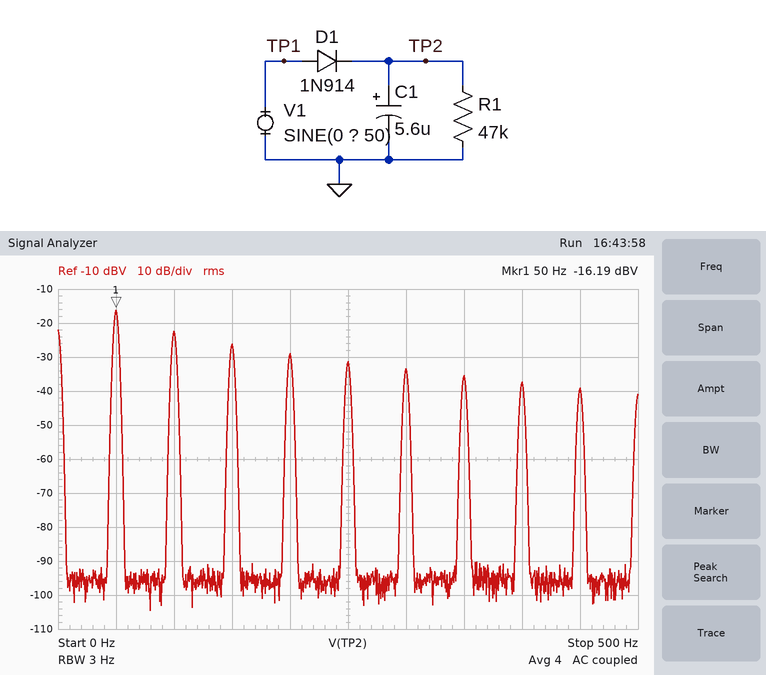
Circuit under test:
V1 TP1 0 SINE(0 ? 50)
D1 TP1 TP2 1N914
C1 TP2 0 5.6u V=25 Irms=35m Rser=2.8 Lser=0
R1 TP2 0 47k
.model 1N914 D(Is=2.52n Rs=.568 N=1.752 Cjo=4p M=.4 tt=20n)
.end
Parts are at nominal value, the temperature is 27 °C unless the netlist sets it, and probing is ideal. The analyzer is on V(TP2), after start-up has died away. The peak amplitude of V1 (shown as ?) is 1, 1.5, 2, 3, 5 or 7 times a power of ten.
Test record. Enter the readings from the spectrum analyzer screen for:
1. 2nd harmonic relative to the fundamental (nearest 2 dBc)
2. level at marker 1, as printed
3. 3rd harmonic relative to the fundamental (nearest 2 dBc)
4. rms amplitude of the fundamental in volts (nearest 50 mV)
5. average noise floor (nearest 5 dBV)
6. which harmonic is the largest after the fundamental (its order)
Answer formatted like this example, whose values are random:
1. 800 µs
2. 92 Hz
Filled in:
1. -6 dBc
2. -16.19 dBV
3. -10 dBc
4. 150 mV
5. -95 dBV
6. 2
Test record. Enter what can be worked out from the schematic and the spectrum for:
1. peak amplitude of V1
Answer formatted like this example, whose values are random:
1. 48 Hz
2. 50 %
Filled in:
1. 10 V
